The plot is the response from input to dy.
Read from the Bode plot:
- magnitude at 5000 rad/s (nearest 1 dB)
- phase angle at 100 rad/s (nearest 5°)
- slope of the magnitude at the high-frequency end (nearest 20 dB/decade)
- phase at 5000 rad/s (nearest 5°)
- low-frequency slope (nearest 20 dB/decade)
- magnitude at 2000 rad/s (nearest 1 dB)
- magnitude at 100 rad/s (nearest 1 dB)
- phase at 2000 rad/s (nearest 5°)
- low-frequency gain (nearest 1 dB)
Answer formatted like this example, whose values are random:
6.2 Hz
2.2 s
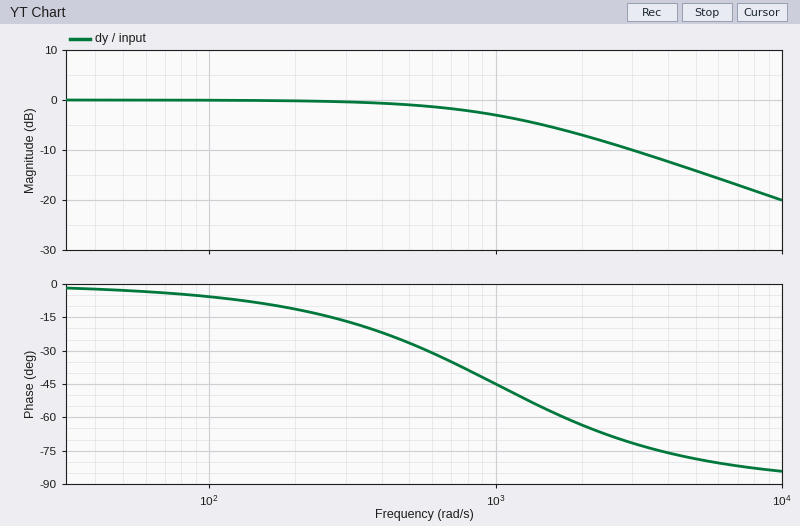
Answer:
-14 dB
-5°
-20 dB/decade
-80°
0 dB/decade
-7 dB
0 dB
-65°
0 dB
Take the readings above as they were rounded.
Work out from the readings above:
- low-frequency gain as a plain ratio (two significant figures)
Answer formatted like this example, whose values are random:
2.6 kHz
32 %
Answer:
1.0
